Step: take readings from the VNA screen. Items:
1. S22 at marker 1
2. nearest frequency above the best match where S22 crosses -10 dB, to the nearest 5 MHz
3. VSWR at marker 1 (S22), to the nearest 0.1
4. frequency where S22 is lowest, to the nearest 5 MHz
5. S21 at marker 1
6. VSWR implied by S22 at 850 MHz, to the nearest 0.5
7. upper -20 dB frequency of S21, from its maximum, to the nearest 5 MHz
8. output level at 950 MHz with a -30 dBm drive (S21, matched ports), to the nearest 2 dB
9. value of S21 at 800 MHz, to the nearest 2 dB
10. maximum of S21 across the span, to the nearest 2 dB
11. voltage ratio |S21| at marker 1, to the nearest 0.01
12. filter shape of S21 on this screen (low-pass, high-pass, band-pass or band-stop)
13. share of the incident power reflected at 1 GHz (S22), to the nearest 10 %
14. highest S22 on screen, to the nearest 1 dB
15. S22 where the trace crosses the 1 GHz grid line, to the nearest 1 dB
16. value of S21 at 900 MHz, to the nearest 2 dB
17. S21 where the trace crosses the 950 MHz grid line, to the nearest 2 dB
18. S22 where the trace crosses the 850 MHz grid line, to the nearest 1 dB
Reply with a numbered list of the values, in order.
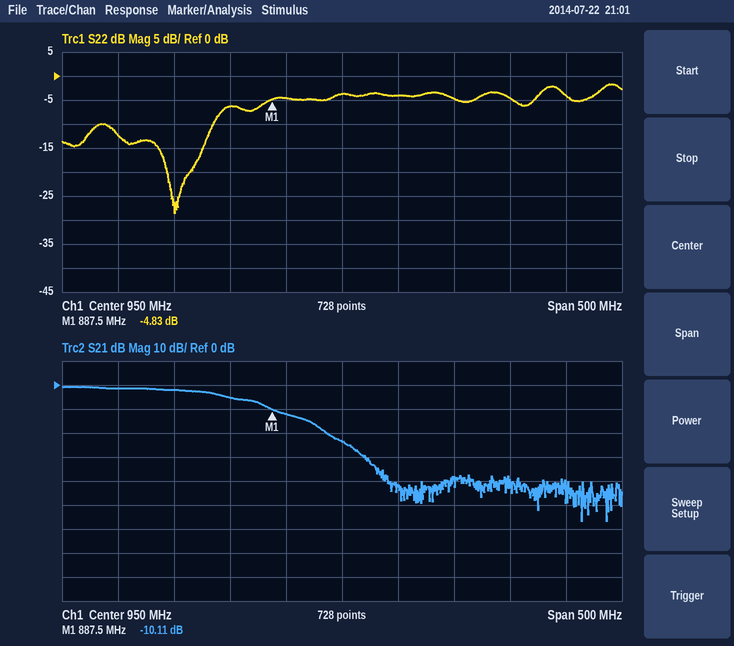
1. -4.83 dB
2. 835 MHz
3. 3.7
4. 800 MHz
5. -10.11 dB
6. 3.0
7. 940 MHz
8. -54 dBm
9. -2 dB
10. 0 dB
11. 0.31
12. low-pass
13. 40 %
14. -2 dB
15. -4 dB
16. -12 dB
17. -24 dB
18. -6 dB
